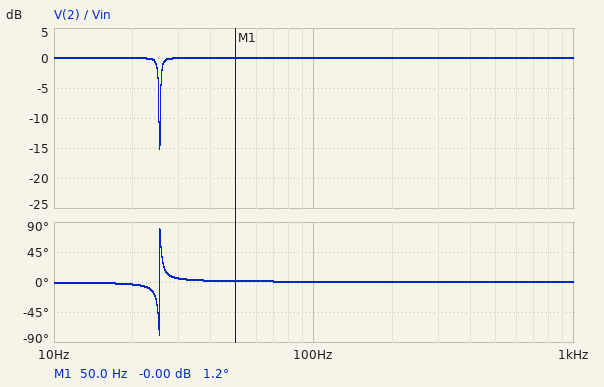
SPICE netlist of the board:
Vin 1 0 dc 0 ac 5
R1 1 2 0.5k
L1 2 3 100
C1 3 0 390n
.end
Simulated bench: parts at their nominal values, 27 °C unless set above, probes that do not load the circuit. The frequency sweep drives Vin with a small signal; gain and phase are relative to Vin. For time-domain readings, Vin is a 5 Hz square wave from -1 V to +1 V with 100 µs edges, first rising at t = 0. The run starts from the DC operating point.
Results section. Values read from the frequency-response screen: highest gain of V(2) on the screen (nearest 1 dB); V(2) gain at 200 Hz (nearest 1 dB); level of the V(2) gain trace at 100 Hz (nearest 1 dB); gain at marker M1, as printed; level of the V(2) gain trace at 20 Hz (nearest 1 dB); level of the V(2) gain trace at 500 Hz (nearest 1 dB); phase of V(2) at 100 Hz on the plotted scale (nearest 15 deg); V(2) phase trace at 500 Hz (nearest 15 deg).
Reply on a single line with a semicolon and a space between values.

0 dB; 0 dB; 0 dB; -0.00 dB; 0 dB; 0 dB; 0 deg; 0 deg
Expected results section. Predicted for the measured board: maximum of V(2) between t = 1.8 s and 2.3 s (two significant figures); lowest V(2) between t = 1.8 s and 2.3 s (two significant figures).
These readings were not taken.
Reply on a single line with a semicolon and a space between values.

1.2 V; -1.2 V
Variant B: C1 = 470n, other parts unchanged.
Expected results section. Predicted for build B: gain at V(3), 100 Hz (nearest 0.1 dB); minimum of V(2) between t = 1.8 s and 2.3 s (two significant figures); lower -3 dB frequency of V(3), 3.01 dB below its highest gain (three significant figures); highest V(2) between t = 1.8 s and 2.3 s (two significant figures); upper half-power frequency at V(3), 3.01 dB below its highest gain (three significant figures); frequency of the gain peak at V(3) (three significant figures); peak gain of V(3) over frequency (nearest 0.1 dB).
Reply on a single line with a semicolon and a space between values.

-24.9 dB; -1.1 V; 22.8 Hz; 1.1 V; 23.6 Hz; 23.2 Hz; 29.3 dB
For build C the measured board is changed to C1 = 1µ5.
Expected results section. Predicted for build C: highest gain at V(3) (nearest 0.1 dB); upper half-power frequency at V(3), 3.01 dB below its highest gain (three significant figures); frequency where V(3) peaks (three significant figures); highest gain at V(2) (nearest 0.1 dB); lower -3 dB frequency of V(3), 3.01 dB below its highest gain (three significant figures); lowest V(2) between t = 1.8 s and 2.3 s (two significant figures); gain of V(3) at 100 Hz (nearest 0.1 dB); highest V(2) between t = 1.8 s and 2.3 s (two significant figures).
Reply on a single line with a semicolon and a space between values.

24.3 dB; 13.4 Hz; 13.0 Hz; 0 dB; 12.6 Hz; -1.1 V; -35.3 dB; 1.1 V
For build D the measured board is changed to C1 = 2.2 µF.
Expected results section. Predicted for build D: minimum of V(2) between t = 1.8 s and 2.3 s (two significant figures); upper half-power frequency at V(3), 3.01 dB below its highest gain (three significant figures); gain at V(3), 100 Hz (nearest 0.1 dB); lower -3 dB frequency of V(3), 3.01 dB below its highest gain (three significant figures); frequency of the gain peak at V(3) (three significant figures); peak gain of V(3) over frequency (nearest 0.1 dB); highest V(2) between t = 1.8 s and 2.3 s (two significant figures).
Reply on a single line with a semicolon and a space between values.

-1.1 V; 11.1 Hz; -38.7 dB; 10.3 Hz; 10.7 Hz; 22.6 dB; 1.1 V
